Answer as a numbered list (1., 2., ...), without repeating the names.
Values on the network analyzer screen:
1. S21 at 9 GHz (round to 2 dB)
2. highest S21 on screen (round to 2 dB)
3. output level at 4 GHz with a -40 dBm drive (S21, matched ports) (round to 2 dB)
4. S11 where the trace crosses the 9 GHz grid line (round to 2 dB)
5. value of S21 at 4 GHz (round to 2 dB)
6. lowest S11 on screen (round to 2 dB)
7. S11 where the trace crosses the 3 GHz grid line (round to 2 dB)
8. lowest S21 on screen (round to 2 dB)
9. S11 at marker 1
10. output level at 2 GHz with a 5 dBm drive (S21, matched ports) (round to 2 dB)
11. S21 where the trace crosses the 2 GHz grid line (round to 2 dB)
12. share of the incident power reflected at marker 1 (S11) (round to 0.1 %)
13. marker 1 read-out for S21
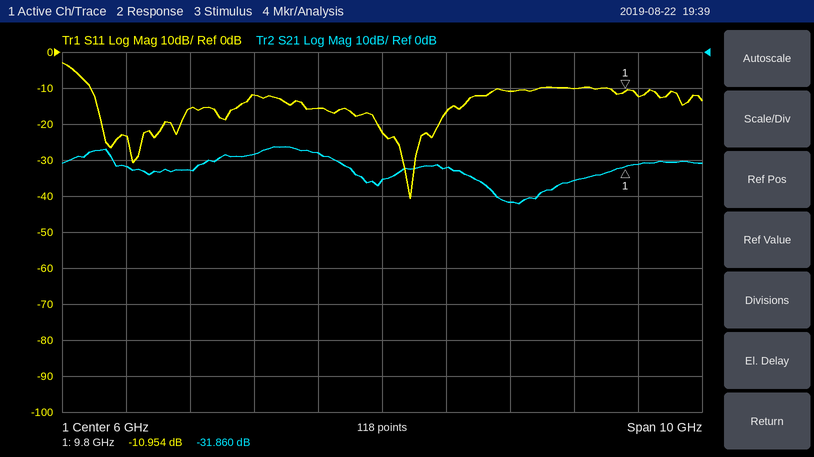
1. -36 dB
2. -26 dB
3. -68 dBm
4. -10 dB
5. -28 dB
6. -40 dB
7. -16 dB
8. -42 dB
9. -10.954 dB
10. -26 dBm
11. -32 dB
12. 8.0 %
13. -31.860 dB
